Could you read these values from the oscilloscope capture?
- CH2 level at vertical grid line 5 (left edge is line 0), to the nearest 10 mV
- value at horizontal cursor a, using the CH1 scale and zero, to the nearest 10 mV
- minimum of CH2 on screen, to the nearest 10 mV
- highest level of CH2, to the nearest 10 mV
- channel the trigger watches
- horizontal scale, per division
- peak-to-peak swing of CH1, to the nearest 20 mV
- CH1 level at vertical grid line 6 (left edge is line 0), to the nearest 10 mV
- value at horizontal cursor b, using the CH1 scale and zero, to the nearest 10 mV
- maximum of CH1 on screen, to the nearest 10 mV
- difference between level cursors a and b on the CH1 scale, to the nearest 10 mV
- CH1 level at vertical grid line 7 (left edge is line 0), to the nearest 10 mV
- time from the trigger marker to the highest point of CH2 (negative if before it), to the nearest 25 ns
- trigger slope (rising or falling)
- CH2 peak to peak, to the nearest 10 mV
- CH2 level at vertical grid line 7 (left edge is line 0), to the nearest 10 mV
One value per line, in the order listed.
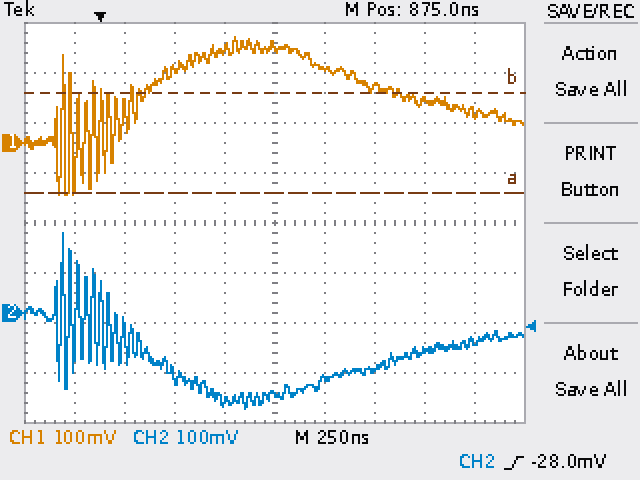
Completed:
-160 mV
-100 mV
-190 mV
160 mV
CH2
250 ns
320 mV
150 mV
100 mV
210 mV
200 mV
110 mV
-175 ns
rising
350 mV
-110 mV
